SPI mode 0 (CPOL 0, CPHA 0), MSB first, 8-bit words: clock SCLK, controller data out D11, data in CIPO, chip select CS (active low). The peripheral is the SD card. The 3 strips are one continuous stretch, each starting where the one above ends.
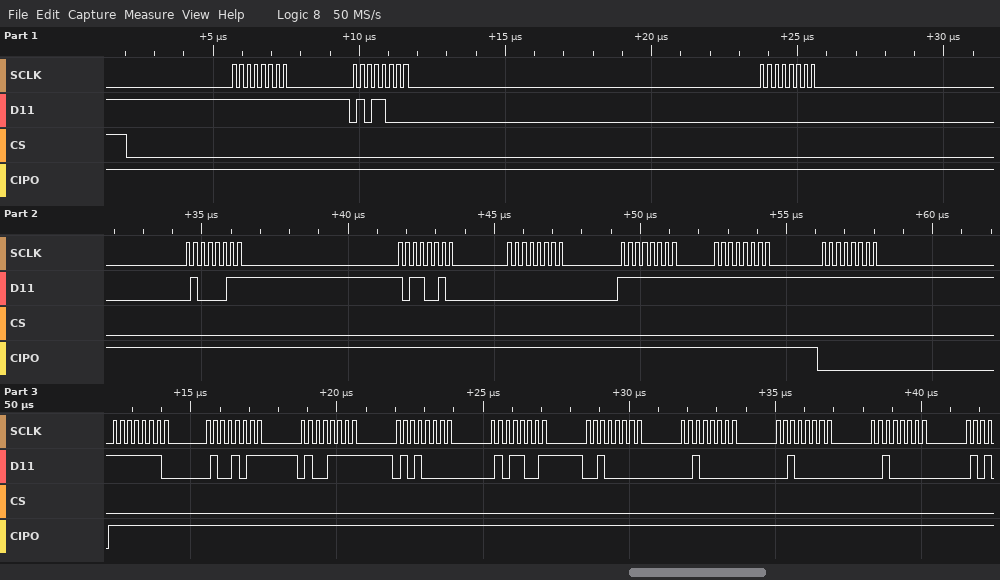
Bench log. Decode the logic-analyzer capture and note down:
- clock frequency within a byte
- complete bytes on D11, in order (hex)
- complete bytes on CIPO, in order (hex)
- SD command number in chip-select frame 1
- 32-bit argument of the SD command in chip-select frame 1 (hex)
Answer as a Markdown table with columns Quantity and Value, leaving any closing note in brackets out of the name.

| Quantity | Value |
|---|---|
| clock frequency within a byte | 4 MHz |
| complete bytes on D11, in order | FF 58 00 43 B2 00 FF FF FF FE 4B 4F 50 59 20 20 20 20 |
| complete bytes on CIPO, in order | FF FF FF FF FF FF FF FF 00 FF FF FF FF FF FF FF FF FF |
| SD command number in chip-select frame 1 | CMD24 |
| 32-bit argument of the SD command in chip-select frame 1 | 0x0043B200 |
